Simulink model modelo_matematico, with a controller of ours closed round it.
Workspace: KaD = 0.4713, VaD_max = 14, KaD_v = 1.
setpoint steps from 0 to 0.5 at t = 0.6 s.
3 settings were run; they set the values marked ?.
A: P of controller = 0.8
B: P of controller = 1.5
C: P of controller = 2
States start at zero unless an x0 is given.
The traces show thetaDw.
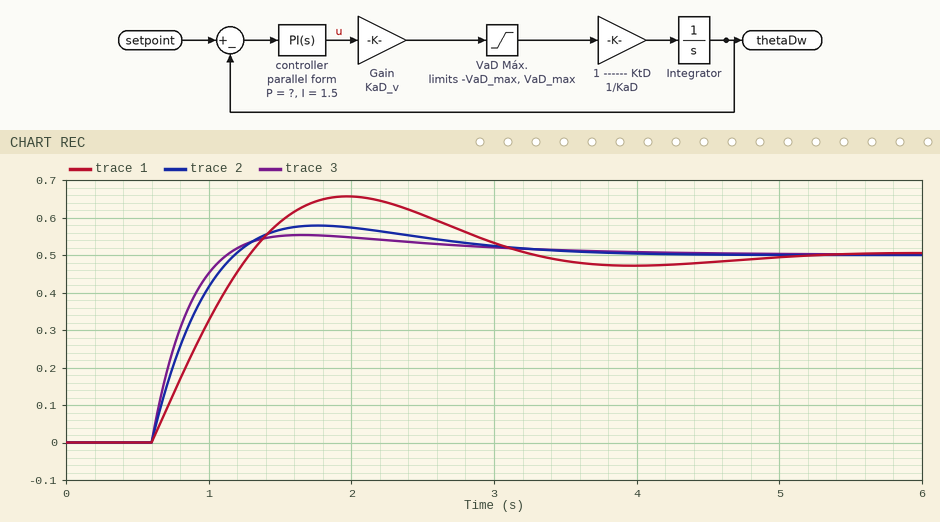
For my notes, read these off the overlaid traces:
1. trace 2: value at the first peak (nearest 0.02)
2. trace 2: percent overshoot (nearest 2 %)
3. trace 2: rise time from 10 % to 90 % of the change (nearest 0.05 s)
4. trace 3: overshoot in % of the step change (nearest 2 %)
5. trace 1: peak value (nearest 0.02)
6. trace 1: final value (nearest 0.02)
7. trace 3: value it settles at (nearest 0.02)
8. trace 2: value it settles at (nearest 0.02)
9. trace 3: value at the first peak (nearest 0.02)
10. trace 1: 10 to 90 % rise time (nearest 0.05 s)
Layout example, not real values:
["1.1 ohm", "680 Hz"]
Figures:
["0.58", "16 %", "0.45 s", "10 %", "0.66", "0.50", "0.50", "0.50", "0.56", "0.55 s"]
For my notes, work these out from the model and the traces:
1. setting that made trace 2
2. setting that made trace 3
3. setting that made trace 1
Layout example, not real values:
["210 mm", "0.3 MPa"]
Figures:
["B", "C", "A"]
